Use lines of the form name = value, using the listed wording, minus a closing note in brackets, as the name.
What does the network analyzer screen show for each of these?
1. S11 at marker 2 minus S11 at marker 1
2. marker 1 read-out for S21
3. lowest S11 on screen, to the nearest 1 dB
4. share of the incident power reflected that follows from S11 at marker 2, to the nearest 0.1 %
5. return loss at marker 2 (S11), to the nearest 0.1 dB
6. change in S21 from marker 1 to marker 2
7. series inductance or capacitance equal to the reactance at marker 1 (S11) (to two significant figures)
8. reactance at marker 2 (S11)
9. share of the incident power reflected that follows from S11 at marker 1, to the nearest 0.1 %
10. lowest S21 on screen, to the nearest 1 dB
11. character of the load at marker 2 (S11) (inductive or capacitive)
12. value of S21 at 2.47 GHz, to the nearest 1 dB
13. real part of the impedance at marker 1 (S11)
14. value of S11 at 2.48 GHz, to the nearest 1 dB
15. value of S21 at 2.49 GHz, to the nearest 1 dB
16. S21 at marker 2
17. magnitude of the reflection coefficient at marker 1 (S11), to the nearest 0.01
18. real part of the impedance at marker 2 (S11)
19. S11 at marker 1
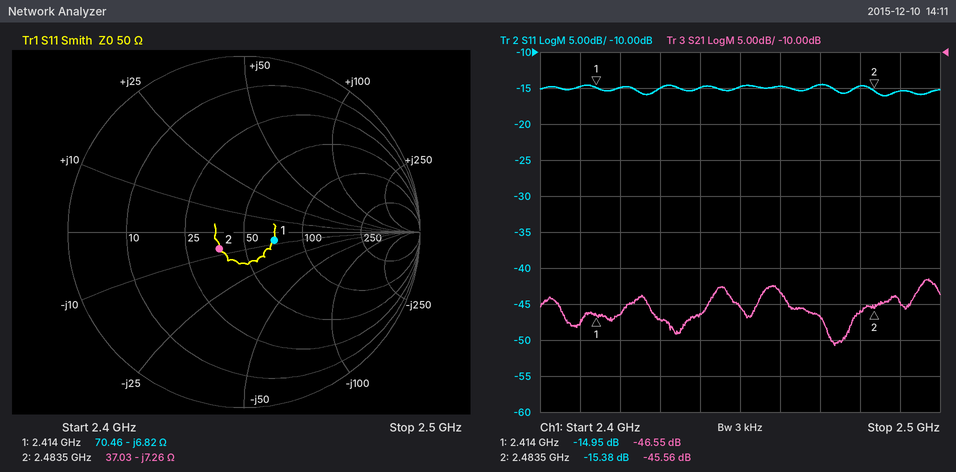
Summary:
S11 at marker 2 minus S11 at marker 1 = -0.43 dB
marker 1 read-out for S21 = -46.55 dB
lowest S11 on screen, to the nearest 1 dB = -16 dB
share of the incident power reflected that follows from S11 at marker 2, to the nearest 0.1 % = 2.9 %
return loss at marker 2 (S11), to the nearest 0.1 dB = 15.4 dB
change in S21 from marker 1 to marker 2 = 0.99 dB
series inductance or capacitance equal to the reactance at marker 1 (S11) = 9.7 pF
reactance at marker 2 = -7.26 Ω
share of the incident power reflected that follows from S11 at marker 1, to the nearest 0.1 % = 3.2 %
lowest S21 on screen, to the nearest 1 dB = -51 dB
character of the load at marker 2 (S11) = capacitive
value of S21 at 2.47 GHz, to the nearest 1 dB = -47 dB
real part of the impedance at marker 1 = 70.46 Ω
value of S11 at 2.48 GHz, to the nearest 1 dB = -15 dB
value of S21 at 2.49 GHz, to the nearest 1 dB = -45 dB
S21 at marker 2 = -45.56 dB
magnitude of the reflection coefficient at marker 1 (S11), to the nearest 0.01 = 0.18
real part of the impedance at marker 2 = 37.03 Ω
S11 at marker 1 = -14.95 dB
